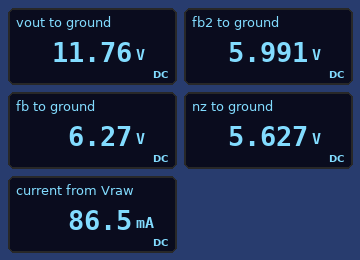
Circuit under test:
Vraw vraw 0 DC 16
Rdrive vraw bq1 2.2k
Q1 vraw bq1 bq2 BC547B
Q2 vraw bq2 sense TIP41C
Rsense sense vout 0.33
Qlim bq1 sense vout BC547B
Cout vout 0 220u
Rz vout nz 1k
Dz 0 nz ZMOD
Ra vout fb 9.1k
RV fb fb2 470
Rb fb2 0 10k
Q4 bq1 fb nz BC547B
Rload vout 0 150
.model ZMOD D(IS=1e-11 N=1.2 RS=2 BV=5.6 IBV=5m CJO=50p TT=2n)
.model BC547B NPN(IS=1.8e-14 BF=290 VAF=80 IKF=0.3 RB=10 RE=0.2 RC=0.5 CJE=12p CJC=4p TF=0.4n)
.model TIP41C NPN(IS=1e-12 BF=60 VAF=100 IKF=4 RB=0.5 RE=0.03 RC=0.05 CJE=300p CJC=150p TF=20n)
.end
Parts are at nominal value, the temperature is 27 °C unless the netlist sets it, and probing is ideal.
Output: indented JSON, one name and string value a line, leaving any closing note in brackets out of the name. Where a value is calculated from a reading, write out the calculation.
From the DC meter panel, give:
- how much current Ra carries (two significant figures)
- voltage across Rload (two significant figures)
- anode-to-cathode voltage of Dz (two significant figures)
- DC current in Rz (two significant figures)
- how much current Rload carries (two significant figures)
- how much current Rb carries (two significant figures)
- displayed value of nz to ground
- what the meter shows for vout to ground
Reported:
{
  "how much current Ra carries": "(11.76 V - 6.27 V) / 9.1 kΩ = 600 µA",
  "voltage across Rload": "11.76 V = 12 V",
  "anode-to-cathode voltage of Dz": "0 V - 5.627 V = -5.6 V",
  "DC current in Rz": "(11.76 V - 5.627 V) / 1 kΩ = 6.1 mA",
  "how much current Rload carries": "(11.76 V) / 150 Ω = 78 mA",
  "how much current Rb carries": "(5.991 V) / 10 kΩ = 600 µA",
  "displayed value of nz to ground": "5.627 V",
  "what the meter shows for vout to ground": "11.76 V"
}
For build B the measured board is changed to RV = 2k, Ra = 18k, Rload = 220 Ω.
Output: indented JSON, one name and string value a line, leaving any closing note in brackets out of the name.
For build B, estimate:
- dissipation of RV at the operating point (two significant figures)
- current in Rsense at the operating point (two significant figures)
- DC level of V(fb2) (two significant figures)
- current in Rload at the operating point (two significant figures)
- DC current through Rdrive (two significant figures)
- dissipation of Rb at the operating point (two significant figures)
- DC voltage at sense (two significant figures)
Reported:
{
  "dissipation of RV at the operating point": "480 µW",
  "current in Rsense at the operating point": "76 mA",
  "DC level of V(fb2)": "4.9 V",
  "current in Rload at the operating point": "67 mA",
  "DC current through Rdrive": "4.4 µA",
  "dissipation of Rb at the operating point": "2.4 mW",
  "DC voltage at sense": "15 V"
}
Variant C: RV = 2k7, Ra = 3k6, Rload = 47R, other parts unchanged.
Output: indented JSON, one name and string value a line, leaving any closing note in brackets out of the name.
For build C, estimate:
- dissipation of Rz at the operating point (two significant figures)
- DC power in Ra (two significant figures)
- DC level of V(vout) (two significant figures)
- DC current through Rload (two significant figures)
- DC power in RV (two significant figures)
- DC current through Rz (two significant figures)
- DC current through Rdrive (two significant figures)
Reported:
{
  "dissipation of Rz at the operating point": "6.2 mW",
  "DC power in Ra": "920 µW",
  "DC level of V(vout)": "8.1 V",
  "DC current through Rload": "170 mA",
  "DC power in RV": "660 µW",
  "DC current through Rz": "2.5 mA",
  "DC current through Rdrive": "3.0 mA"
}
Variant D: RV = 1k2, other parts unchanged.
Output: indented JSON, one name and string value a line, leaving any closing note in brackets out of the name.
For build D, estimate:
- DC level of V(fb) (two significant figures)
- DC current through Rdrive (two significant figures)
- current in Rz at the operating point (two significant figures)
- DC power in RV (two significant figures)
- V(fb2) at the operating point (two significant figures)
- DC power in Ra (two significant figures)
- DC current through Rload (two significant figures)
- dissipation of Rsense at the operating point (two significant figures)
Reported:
{
  "DC level of V(fb)": "6.3 V",
  "DC current through Rdrive": "1.5 mA",
  "current in Rz at the operating point": "5.8 mA",
  "DC power in RV": "380 µW",
  "V(fb2) at the operating point": "5.6 V",
  "DC power in Ra": "2.9 mW",
  "DC current through Rload": "76 mA",
  "dissipation of Rsense at the operating point": "2.2 mW"
}
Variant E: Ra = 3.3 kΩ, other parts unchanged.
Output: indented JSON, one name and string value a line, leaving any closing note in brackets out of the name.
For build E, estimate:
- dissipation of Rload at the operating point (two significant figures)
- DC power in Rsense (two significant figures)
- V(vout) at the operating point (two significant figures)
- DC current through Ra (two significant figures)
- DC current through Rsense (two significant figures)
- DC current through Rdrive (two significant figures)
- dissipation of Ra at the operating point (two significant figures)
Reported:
{
  "dissipation of Rload at the operating point": "460 mW",
  "DC power in Rsense": "1.1 mW",
  "V(vout) at the operating point": "8.3 V",
  "DC current through Ra": "610 µA",
  "DC current through Rsense": "59 mA",
  "DC current through Rdrive": "2.9 mA",
  "dissipation of Ra at the operating point": "1.2 mW"
}
